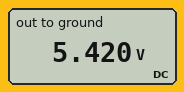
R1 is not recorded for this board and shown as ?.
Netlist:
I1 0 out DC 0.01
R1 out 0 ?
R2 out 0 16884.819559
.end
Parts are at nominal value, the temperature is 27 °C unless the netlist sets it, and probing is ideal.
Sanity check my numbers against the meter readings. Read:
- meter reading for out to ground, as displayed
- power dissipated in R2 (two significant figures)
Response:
5.420 V
1.7 mW
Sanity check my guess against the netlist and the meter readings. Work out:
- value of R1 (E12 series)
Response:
560 Ω
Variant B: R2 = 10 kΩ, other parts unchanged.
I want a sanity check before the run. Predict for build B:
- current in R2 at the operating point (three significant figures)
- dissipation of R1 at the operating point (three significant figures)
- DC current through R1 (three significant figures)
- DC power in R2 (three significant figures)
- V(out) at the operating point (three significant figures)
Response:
530 µA
50.2 mW
9.47 mA
2.81 mW
5.30 V
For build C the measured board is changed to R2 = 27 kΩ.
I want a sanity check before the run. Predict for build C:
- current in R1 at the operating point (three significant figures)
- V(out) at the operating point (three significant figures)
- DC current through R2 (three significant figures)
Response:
9.80 mA
5.49 V
203 µA
